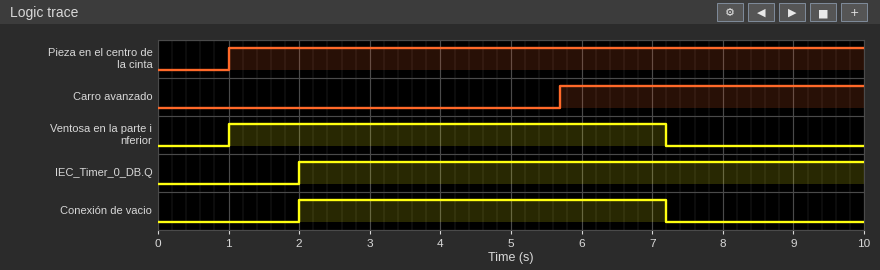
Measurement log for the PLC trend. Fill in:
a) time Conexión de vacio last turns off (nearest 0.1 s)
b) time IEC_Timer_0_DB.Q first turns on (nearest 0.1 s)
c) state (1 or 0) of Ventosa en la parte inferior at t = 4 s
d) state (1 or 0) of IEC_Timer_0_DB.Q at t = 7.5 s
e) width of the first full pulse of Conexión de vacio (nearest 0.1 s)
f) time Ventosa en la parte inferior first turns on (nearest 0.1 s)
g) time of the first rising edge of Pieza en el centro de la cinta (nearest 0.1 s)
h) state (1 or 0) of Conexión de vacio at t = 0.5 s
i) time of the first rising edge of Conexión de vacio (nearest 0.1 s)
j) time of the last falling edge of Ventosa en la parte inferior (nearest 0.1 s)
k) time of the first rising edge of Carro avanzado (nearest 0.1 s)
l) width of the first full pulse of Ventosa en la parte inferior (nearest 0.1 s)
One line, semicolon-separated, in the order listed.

7.2 s; 2.0 s; 1; 1; 5.2 s; 1.0 s; 1.0 s; 0; 2.0 s; 7.2 s; 5.7 s; 6.2 s
